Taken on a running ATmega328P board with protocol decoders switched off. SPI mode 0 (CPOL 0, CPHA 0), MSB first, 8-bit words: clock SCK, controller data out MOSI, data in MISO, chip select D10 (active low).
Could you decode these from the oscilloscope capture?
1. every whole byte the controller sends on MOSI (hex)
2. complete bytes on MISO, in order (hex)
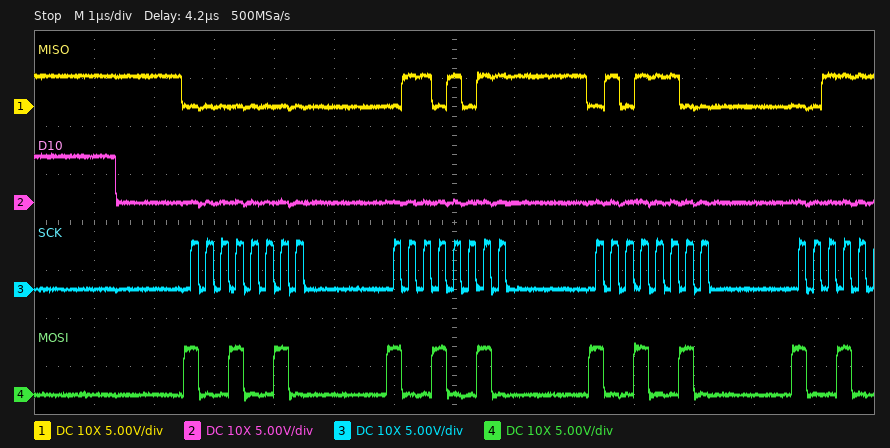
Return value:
0x92 0x92 0x92
0x00 0x6B 0x5C
